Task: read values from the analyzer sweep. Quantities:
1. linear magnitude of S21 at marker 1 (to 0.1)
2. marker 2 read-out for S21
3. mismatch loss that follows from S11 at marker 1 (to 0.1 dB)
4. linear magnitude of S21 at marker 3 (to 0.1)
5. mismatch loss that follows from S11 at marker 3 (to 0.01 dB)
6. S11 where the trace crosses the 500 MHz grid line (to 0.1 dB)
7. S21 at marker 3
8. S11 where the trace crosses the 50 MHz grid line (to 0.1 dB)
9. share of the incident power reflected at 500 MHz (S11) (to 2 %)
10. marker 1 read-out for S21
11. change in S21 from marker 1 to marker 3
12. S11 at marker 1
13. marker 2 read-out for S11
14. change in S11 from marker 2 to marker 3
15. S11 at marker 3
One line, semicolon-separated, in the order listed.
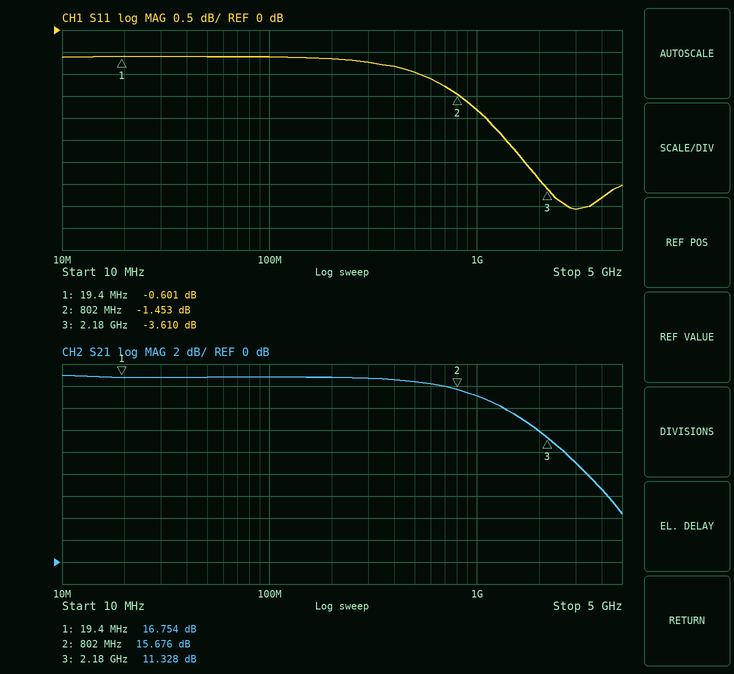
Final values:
6.9; 15.676 dB; 8.9 dB; 3.7; 2.48 dB; -1.0 dB; 11.328 dB; -0.6 dB; 80 %; 16.754 dB; -5.426 dB; -0.601 dB; -1.453 dB; -2.157 dB; -3.610 dB
